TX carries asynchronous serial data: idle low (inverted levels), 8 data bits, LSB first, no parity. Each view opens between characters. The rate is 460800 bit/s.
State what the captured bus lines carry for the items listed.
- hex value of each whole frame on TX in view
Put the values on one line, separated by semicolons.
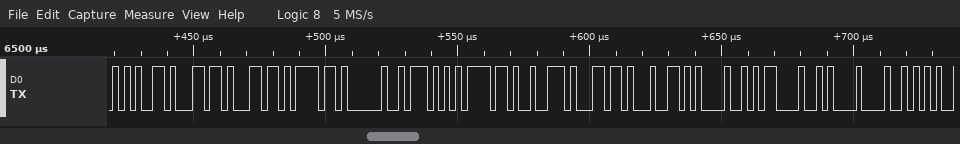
35, 27, 27, 21, BF, 51, 21, 1B, 27, 37, BD, E5, EB, 6F
